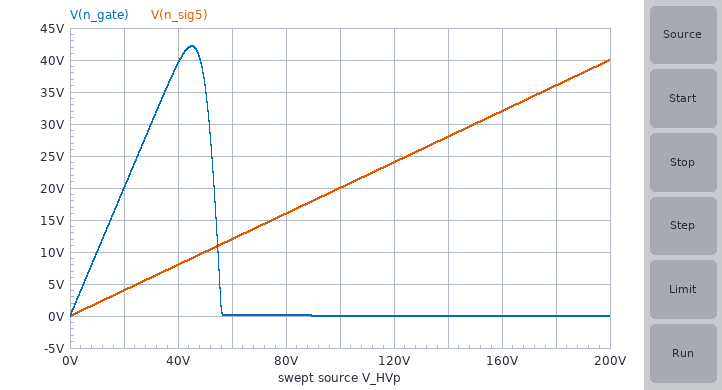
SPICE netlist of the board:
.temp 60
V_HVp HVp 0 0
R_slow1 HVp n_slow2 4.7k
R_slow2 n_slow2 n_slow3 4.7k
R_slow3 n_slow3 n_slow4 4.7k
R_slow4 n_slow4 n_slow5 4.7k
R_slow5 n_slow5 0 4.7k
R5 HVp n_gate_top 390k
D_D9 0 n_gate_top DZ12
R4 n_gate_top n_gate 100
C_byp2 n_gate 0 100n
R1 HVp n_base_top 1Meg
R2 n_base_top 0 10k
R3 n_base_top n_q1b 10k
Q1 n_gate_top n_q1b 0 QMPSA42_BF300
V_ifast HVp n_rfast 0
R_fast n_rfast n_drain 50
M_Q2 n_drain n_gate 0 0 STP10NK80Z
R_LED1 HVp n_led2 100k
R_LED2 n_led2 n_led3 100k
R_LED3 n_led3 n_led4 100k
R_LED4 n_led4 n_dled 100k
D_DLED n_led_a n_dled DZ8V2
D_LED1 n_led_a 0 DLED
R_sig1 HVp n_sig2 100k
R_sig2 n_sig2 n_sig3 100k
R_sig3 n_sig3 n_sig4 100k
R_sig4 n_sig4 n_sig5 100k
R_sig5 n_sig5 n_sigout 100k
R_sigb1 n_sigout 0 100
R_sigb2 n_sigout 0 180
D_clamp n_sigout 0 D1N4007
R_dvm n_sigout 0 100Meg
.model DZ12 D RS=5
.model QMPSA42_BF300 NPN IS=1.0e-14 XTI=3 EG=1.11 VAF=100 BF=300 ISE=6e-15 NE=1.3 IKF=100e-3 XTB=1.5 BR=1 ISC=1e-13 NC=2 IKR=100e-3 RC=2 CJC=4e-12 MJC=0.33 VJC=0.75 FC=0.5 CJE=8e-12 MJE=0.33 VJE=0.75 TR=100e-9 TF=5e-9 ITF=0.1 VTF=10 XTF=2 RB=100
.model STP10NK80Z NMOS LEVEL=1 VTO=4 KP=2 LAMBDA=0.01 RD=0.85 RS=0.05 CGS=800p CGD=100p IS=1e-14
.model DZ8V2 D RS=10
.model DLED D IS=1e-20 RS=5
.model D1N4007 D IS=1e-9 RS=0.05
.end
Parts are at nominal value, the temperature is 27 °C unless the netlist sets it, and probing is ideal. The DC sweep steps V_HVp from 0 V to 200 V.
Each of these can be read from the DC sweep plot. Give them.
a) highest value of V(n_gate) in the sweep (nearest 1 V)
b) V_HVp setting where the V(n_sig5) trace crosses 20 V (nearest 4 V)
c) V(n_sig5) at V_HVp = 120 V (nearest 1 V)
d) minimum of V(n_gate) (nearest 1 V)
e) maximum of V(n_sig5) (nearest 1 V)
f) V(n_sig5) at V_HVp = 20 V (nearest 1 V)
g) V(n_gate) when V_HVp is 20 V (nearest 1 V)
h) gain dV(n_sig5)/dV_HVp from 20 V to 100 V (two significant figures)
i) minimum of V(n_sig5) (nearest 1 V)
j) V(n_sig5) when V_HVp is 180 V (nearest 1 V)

42 V
100 V
24 V
0 V
40 V
4 V
20 V
0.20 V/V
0 V
36 V
